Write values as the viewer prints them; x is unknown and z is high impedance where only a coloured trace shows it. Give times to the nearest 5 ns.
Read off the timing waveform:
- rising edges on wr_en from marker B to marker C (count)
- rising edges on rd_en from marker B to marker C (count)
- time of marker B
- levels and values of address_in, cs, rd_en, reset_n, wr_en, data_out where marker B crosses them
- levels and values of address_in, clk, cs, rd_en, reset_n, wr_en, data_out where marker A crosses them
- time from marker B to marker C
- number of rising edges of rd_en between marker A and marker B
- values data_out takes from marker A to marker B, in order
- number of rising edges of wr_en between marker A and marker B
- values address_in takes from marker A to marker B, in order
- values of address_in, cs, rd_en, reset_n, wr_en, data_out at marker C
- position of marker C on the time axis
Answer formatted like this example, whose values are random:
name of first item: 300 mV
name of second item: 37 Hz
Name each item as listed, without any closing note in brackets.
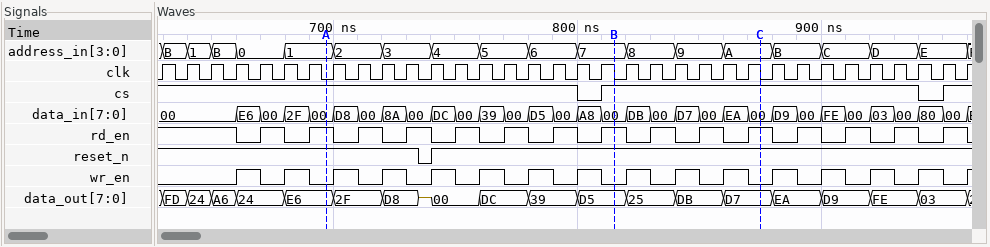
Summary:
rising edges on wr_en from marker B to marker C: 3
rising edges on rd_en from marker B to marker C: 3
time of marker B: 815 ns
levels and values of address_in, cs, rd_en, reset_n, wr_en, data_out where marker B crosses them: address_in=7, cs=1, rd_en=1, reset_n=1, wr_en=0, data_out=D5
levels and values of address_in, clk, cs, rd_en, reset_n, wr_en, data_out where marker A crosses them: address_in=1, clk=0, cs=1, rd_en=1, reset_n=1, wr_en=0, data_out=E6
time from marker B to marker C: 60 ns
number of rising edges of rd_en between marker A and marker B: 6
values data_out takes from marker A to marker B, in order: E6, 2F, D8, z, 00, DC, 39, D5
number of rising edges of wr_en between marker A and marker B: 6
values address_in takes from marker A to marker B, in order: 1, 2, 3, 4, 5, 6, 7
values of address_in, cs, rd_en, reset_n, wr_en, data_out at marker C: address_in=A, cs=1, rd_en=1, reset_n=1, wr_en=0, data_out=D7
position of marker C on the time axis: 875 ns
